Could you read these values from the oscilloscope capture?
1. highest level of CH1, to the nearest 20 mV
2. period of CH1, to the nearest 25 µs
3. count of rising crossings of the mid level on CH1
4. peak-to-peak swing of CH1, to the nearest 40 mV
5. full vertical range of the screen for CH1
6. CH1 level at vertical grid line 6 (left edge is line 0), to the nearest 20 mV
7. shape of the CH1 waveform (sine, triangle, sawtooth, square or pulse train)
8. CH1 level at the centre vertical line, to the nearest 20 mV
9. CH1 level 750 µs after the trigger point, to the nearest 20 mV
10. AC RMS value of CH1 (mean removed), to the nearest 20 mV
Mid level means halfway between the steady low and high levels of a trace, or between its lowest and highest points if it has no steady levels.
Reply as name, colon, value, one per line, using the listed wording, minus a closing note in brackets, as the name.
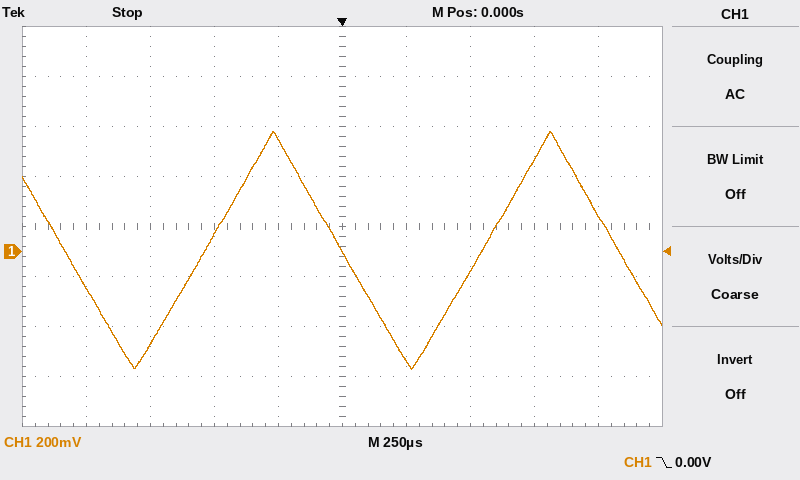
highest level of CH1, to the nearest 20 mV: 480 mV
period of CH1, to the nearest 25 µs: 1.075 ms
count of rising crossings of the mid level on CH1: 2
peak-to-peak swing of CH1, to the nearest 40 mV: 960 mV
full vertical range of the screen for CH1: 1.6 V
CH1 level at vertical grid line 6 (left edge is line 0), to the nearest 20 mV: -440 mV
shape of the CH1 waveform: triangle
CH1 level at the centre vertical line, to the nearest 20 mV: 0 mV
CH1 level 750 µs after the trigger point, to the nearest 20 mV: 360 mV
AC RMS value of CH1 (mean removed), to the nearest 20 mV: 280 mV
